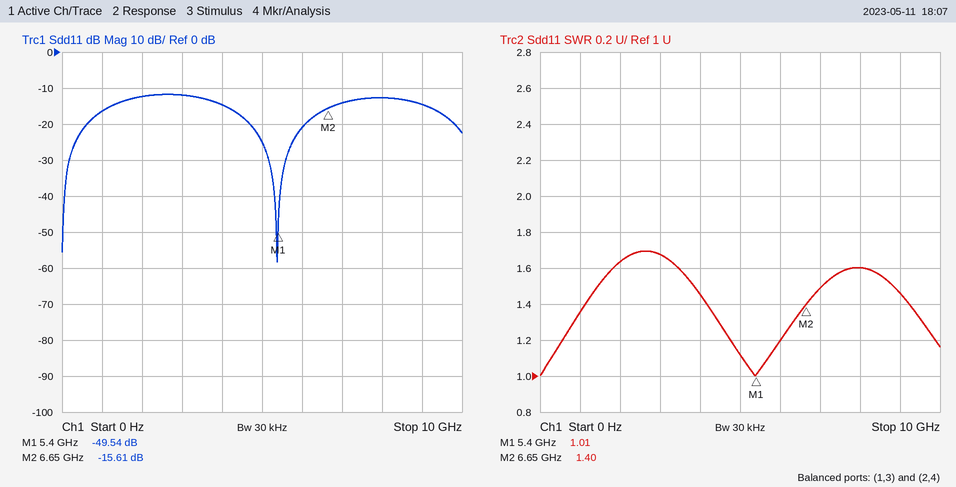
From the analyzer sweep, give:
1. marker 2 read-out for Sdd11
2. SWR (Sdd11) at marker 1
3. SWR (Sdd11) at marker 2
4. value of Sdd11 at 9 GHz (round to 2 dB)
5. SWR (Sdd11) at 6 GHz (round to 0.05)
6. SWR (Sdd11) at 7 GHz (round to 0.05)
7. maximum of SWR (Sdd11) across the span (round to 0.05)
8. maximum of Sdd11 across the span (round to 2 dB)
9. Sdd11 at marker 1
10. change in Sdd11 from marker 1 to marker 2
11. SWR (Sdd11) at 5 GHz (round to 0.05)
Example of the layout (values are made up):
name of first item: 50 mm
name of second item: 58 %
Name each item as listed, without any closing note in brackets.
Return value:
marker 2 read-out for Sdd11: -15.61 dB
SWR (Sdd11) at marker 1: 1.01
SWR (Sdd11) at marker 2: 1.40
value of Sdd11 at 9 GHz: -14 dB
SWR (Sdd11) at 6 GHz: 1.20
SWR (Sdd11) at 7 GHz: 1.50
maximum of SWR (Sdd11) across the span: 1.70
maximum of Sdd11 across the span: -12 dB
Sdd11 at marker 1: -49.54 dB
change in Sdd11 from marker 1 to marker 2: 33.93 dB
SWR (Sdd11) at 5 GHz: 1.10
